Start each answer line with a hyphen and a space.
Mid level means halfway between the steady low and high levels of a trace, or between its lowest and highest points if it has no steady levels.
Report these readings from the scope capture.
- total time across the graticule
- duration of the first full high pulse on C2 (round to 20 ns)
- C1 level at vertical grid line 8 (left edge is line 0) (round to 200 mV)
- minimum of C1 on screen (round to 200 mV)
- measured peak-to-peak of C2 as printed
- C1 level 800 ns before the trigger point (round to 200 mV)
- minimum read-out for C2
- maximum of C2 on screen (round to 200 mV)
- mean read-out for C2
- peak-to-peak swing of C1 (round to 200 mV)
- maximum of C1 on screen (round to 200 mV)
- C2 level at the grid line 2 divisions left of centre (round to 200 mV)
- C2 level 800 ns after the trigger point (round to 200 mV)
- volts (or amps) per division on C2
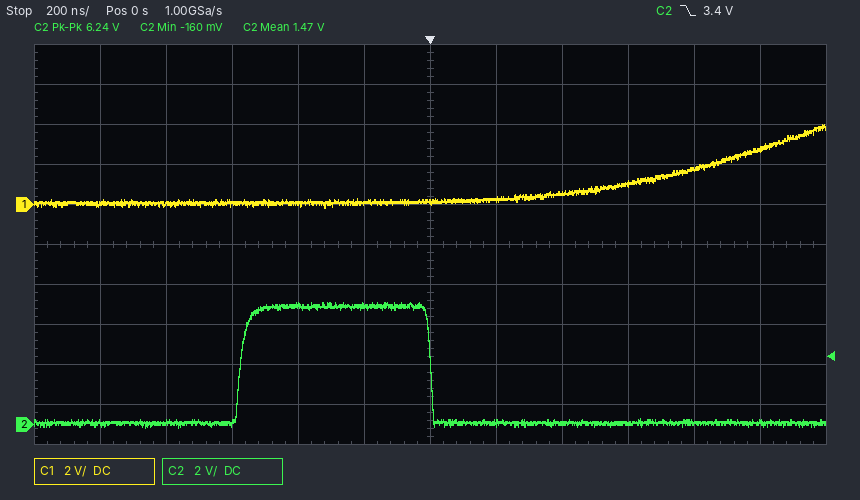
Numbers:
- 2.4 µs
- 580 ns
- 600 mV
- -200 mV
- 6.24 V
- 0.0 V
- -160 mV
- 6.0 V
- 1.47 V
- 4.2 V
- 4.0 V
- 6.0 V
- 200 mV
- 2 V
